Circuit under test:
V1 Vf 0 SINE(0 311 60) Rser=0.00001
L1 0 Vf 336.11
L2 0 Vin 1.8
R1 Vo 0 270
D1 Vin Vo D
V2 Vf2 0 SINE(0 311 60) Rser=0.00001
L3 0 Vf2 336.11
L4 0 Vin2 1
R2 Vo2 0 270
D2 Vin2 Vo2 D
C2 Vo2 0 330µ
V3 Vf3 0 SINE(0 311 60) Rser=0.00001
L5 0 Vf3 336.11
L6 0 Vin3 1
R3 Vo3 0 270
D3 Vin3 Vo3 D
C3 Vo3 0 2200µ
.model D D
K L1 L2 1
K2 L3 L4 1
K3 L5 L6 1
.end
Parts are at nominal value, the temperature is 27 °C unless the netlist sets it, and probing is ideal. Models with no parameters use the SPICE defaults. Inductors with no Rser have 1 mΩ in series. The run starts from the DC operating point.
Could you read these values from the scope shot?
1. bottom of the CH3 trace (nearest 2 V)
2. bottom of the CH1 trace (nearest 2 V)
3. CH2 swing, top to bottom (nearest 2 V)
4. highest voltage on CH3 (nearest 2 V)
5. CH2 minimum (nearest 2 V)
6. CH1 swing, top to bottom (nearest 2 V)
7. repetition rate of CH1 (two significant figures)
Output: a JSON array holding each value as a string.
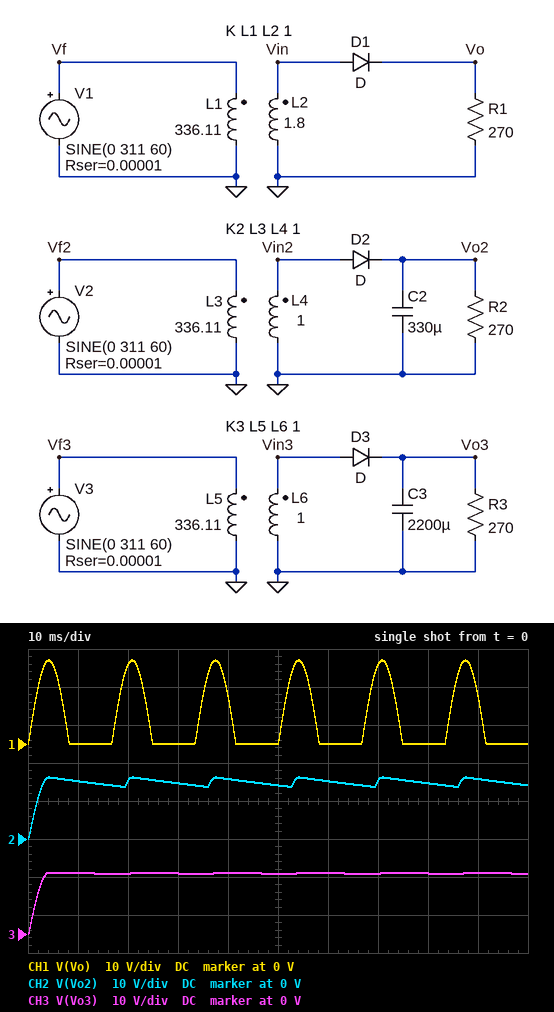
["0 V", "0 V", "16 V", "16 V", "0 V", "22 V", "60 Hz"]
